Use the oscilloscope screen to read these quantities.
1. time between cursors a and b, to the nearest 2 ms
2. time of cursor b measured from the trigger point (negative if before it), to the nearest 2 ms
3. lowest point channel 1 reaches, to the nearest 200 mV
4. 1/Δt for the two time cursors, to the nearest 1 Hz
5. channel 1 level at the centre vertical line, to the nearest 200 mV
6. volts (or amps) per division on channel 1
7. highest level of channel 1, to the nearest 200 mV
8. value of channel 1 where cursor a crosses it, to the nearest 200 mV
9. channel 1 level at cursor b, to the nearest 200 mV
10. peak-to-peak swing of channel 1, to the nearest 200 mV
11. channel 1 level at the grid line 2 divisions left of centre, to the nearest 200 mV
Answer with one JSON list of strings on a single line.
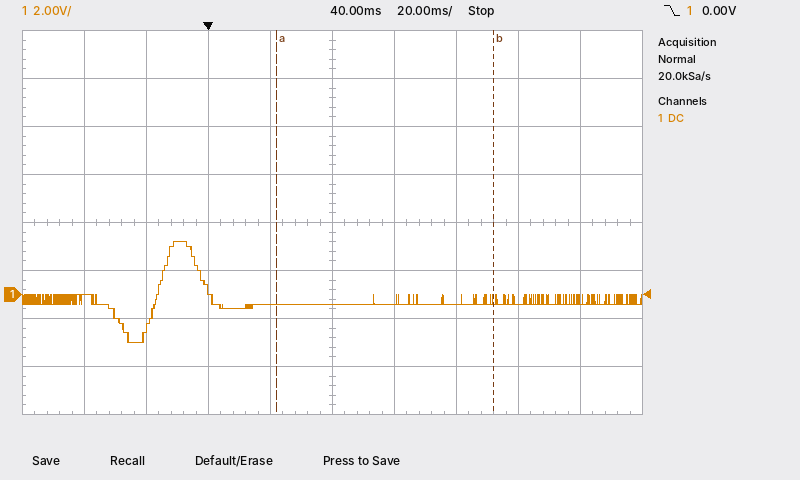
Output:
["70 ms", "+92 ms", "-2.0 V", "14 Hz", "-400 mV", "2 V", "2.2 V", "-400 mV", "-200 mV", "4.2 V", "200 mV"]
